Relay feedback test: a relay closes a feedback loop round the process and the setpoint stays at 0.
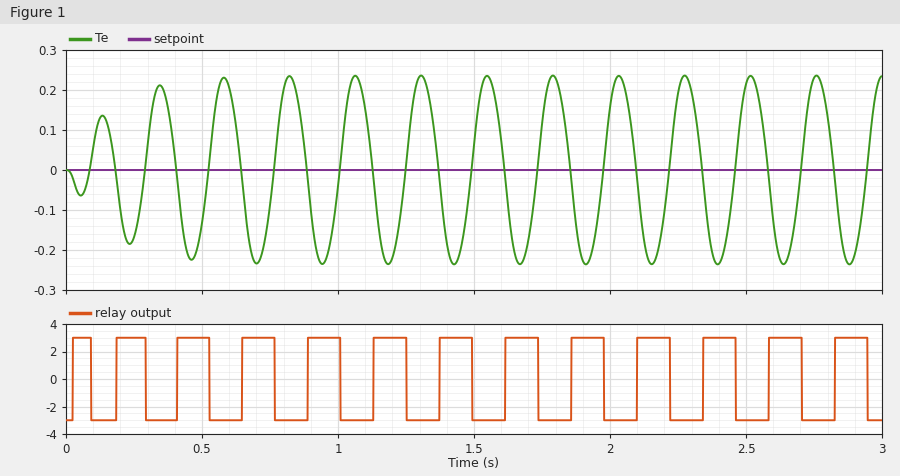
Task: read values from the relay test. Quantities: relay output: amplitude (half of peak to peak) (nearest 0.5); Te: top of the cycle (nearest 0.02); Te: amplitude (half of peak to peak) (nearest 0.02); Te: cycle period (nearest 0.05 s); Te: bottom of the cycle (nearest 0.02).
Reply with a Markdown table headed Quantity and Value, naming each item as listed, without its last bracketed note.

| Quantity | Value |
|---|---|
| relay output: amplitude (half of peak to peak) | 3.0 |
| Te: top of the cycle | 0.24 |
| Te: amplitude (half of peak to peak) | 0.24 |
| Te: cycle period | 0.25 s |
| Te: bottom of the cycle | -0.24 |
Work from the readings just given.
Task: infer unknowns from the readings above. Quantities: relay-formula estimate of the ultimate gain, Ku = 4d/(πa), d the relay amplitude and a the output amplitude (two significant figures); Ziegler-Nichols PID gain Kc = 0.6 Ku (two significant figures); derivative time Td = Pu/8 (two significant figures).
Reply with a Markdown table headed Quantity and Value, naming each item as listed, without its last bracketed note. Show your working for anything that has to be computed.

| Quantity | Value |
|---|---|
| relay-formula estimate of the ultimate gain, Ku = 4d/(πa), d the relay amplitude and a the output amplitude | 4 × 3 / (π × 0.24) = 16 |
| Ziegler-Nichols PID gain Kc = 0.6 Ku | 0.6 × 16 = 9.6 |
| derivative time Td = Pu/8 | 0.25 / 8 = 0.031 s |
